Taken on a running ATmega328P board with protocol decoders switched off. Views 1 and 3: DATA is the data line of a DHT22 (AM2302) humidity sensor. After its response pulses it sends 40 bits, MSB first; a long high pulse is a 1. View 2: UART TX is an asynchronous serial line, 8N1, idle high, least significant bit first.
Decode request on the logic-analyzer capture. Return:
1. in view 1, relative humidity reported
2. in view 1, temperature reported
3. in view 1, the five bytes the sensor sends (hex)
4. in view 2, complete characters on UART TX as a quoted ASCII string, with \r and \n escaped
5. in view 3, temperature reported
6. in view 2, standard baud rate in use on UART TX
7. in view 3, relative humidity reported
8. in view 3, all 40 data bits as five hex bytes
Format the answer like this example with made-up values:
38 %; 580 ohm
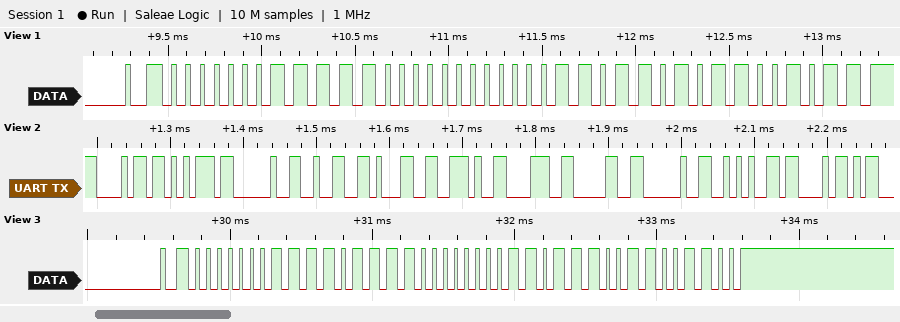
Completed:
49.6 %; 21.8 °C; 01 F0 00 DA CB; "hu 21.80 *C"; 22.0 °C; 115200 baud; 49.5 %; 01 EF 00 DC CC
